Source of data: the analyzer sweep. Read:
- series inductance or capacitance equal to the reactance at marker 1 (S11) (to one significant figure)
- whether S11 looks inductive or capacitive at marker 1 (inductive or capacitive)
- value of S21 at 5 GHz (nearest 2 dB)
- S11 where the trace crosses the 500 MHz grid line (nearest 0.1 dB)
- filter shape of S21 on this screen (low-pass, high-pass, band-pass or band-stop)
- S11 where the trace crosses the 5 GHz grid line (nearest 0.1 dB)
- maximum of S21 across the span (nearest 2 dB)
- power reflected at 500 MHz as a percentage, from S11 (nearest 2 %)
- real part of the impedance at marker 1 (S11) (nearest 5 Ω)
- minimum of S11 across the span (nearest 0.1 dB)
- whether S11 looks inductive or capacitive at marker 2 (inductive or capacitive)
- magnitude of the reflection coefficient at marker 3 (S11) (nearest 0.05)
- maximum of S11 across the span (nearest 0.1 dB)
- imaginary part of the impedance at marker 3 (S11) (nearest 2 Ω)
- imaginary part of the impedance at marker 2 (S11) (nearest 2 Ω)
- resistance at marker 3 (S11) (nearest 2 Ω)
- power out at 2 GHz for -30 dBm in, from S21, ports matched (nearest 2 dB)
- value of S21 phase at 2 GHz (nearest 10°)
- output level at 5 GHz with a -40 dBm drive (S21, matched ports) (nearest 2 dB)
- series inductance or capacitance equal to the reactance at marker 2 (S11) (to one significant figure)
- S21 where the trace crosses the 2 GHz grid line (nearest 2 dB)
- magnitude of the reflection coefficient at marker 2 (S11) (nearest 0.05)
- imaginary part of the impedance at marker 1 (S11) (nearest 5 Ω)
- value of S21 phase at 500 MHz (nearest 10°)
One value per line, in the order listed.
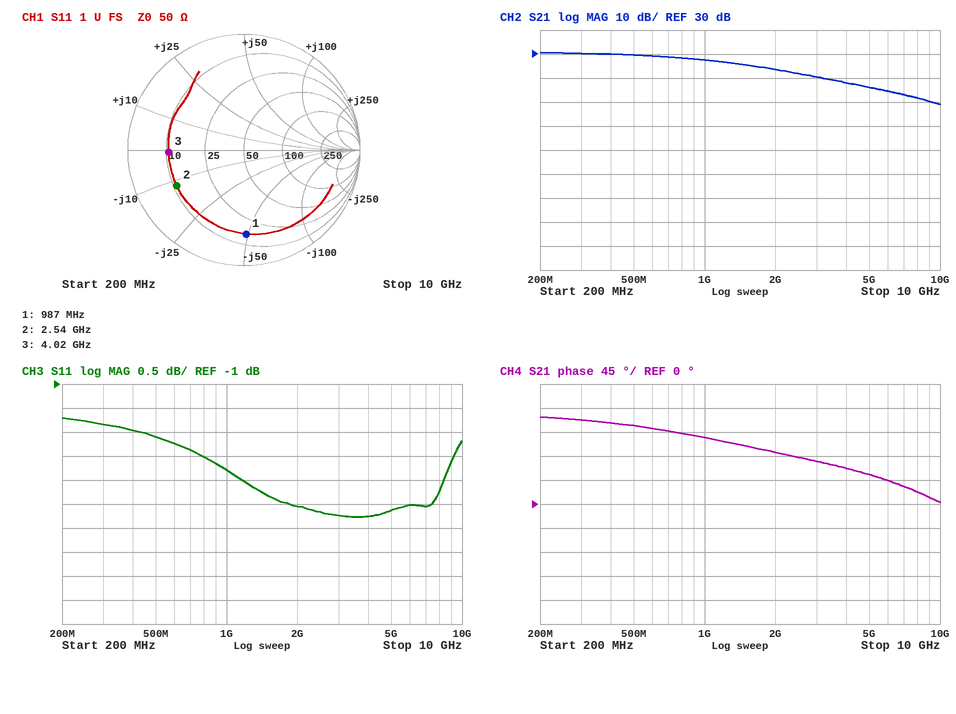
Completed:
3 pF
capacitive
16 dB
-2.1 dB
low-pass
-3.6 dB
30 dB
62 %
15 Ω
-3.8 dB
capacitive
0.65
-1.7 dB
0 Ω
-12 Ω
10 Ω
-6 dBm
100°
-24 dBm
5 pF
24 dB
0.65
-50 Ω
150°
